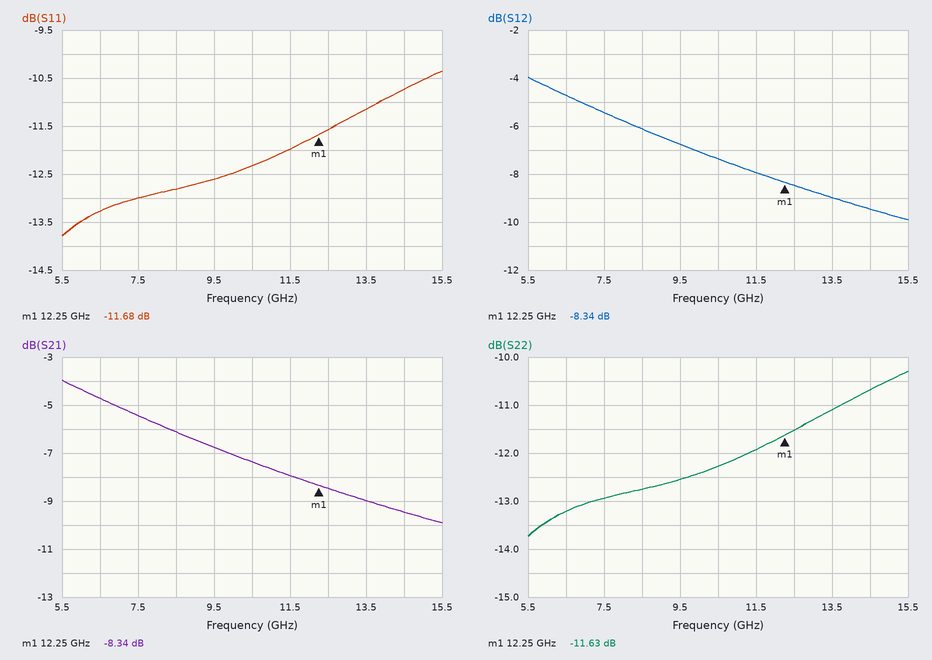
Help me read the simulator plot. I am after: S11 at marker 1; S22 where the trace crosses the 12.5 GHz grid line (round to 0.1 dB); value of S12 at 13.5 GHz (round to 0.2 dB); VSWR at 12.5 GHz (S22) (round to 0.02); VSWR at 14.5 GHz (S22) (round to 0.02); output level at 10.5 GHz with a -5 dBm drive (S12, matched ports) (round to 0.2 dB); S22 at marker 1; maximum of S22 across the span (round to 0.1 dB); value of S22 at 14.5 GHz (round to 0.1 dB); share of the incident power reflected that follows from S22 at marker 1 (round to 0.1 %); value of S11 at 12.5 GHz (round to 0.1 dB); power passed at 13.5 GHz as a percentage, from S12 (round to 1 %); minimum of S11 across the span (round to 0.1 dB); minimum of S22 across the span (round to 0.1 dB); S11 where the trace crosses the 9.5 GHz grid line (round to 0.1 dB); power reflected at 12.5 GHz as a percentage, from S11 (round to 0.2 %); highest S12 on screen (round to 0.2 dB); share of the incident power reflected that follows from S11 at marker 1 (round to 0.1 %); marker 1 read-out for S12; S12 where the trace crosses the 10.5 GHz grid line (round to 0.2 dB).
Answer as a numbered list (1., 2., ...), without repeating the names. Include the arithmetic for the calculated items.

1. -11.68 dB
2. -11.5 dB
3. -9.0 dB
4. |Γ| = 10^(-11.5/20) = 0.2661; VSWR = (1 + 0.2661)/(1 − 0.2661) ≈ 1.73, so 1.72 to the nearest 0.02
5. |Γ| = 10^(-10.7/20) = 0.2917; VSWR = (1 + 0.2917)/(1 − 0.2917) ≈ 1.82
6. -5 dBm + (-7.4 dB) = -12.4 dBm
7. -11.63 dB
8. -10.3 dB
9. -10.7 dB
10. 10^(-11.63/10) ≈ 6.9 %
11. -11.6 dB
12. 10^(-9/10) ≈ 13 %
13. -13.8 dB
14. -13.7 dB
15. -12.6 dB
16. 10^(-11.6/10) ≈ 6.92 %, so 7.0 % to the nearest 0.2 %
17. -4.0 dB
18. 10^(-11.68/10) ≈ 6.8 %
19. -8.34 dB
20. -7.4 dB
